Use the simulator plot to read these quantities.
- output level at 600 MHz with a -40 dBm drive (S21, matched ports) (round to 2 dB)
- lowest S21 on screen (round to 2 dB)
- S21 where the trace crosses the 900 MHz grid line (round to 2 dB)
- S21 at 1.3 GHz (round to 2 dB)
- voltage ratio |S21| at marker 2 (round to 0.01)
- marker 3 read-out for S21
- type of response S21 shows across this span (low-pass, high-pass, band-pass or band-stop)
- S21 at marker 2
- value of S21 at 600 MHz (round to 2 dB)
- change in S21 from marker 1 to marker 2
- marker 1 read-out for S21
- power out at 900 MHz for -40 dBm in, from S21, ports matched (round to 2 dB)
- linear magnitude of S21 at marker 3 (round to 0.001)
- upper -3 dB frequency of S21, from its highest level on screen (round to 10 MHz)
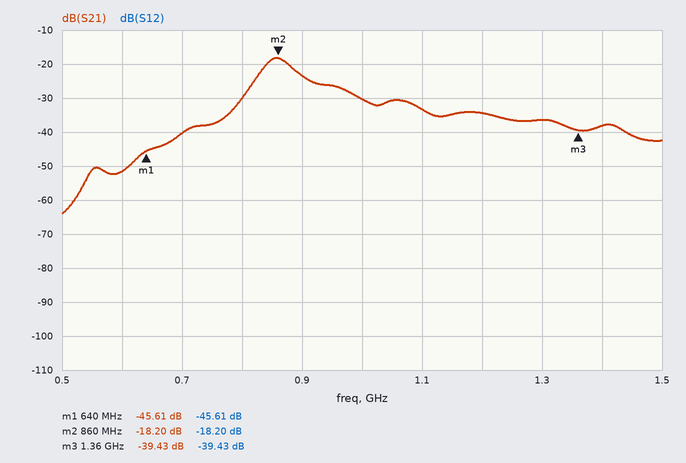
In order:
-92 dBm
-64 dB
-24 dB
-36 dB
0.12
-39.43 dB
band-pass
-18.20 dB
-52 dB
27.41 dB
-45.61 dB
-64 dBm
0.011
880 MHz
